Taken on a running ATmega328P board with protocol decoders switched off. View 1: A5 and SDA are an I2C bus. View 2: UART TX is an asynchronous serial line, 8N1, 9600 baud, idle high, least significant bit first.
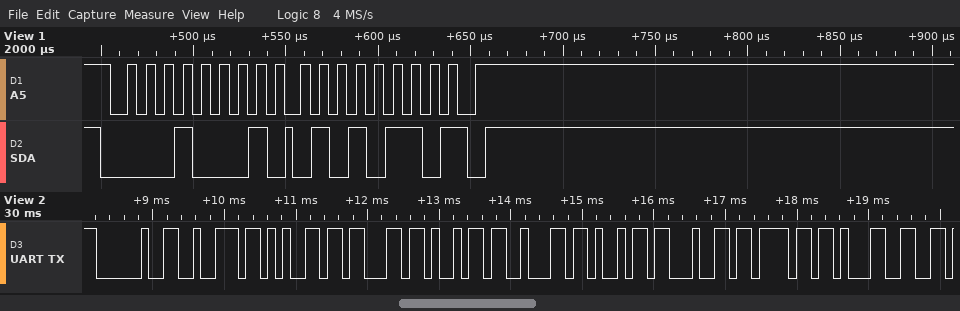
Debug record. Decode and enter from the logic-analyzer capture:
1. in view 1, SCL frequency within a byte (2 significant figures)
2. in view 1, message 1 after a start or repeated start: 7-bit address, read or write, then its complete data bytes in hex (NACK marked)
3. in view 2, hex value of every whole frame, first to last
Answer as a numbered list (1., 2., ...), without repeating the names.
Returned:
1. 100 kHz
2. 0x08 read: 56 NACK
3. 20 72 65 63 69 62 69 64 6F 31
